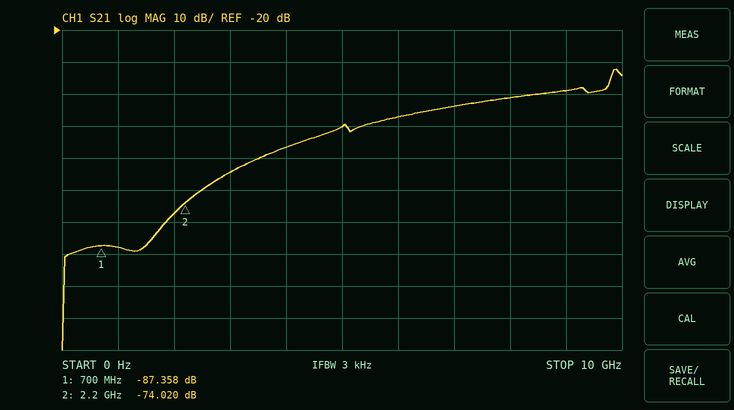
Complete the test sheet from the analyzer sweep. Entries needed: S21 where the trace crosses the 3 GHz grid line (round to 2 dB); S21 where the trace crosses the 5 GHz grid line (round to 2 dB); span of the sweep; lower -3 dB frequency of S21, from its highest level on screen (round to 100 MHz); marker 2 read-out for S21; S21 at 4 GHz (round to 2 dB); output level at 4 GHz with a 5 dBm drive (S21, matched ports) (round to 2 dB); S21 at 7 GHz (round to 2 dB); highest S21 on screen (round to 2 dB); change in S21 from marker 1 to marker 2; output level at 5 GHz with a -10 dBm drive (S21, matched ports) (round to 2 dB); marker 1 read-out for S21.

-64 dB
-50 dB
10 GHz
9.8 GHz
-74.020 dB
-56 dB
-52 dBm
-44 dB
-32 dB
13.338 dB
-60 dBm
-87.358 dB
